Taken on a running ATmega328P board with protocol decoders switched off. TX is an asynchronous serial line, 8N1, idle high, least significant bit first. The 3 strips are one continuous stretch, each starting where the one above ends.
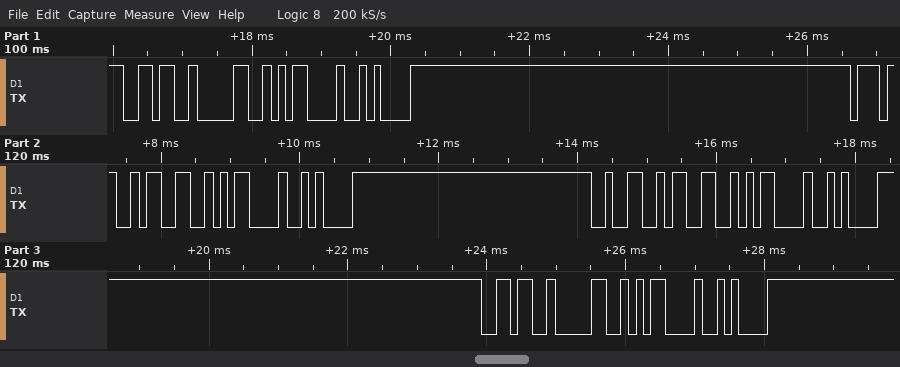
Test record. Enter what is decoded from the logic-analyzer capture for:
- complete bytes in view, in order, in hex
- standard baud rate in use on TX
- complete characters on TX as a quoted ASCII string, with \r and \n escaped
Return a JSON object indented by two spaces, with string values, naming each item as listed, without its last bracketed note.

{
  "complete bytes in view, in order, in hex": "0x36 0x30 0x0D 0x0A 0x37 0x33 0x0D 0x0A 0x32 0x33 0x0D 0x0A 0x36 0x30 0x0D 0x0A",
  "standard baud rate in use on TX": "9600 baud",
  "complete characters on TX as a quoted ASCII string, with \\r and \\n escaped": "\"60\\r\\n73\\r\\n23\\r\\n60\\r\\n\""
}
